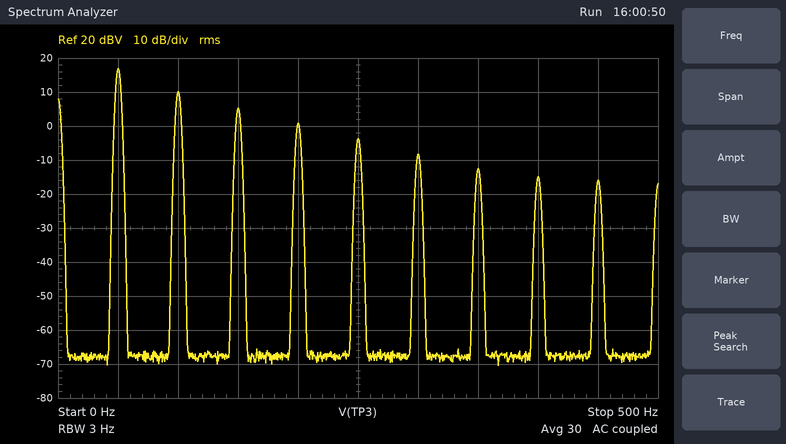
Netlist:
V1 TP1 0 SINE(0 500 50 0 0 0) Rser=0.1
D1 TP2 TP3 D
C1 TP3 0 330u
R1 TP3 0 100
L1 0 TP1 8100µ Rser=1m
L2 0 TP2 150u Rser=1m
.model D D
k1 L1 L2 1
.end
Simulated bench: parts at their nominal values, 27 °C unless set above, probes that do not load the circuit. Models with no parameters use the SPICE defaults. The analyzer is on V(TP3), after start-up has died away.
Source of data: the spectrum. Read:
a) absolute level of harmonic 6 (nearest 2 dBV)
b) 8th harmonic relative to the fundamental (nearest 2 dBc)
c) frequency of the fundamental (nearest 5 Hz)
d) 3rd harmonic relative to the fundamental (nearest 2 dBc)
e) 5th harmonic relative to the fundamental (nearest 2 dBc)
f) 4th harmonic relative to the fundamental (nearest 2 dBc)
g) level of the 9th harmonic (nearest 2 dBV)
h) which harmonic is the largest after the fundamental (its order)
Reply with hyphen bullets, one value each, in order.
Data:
- -8 dBV
- -32 dBc
- 50 Hz
- -12 dBc
- -20 dBc
- -16 dBc
- -16 dBV
- 2
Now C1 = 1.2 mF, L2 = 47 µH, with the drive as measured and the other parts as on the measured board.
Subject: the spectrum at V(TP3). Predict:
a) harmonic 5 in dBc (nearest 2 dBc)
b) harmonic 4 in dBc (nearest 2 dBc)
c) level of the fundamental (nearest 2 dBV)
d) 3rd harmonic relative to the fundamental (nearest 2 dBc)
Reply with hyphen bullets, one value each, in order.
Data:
- -16 dBc
- -14 dBc
- 2 dBV
- -10 dBc
